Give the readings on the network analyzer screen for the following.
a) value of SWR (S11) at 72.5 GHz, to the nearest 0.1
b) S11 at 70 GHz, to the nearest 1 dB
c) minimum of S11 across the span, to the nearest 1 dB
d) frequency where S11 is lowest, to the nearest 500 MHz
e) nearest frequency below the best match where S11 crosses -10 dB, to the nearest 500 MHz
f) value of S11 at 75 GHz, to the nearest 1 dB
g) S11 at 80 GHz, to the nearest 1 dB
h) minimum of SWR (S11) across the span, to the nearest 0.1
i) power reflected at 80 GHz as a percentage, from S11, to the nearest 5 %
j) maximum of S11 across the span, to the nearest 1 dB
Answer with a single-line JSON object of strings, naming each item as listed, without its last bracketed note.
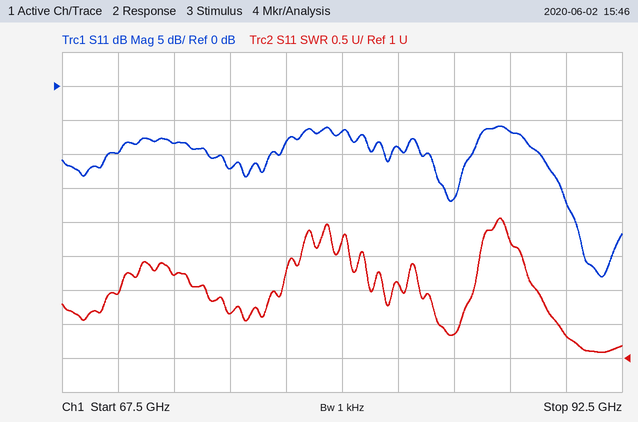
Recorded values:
{"value of SWR (S11) at 72.5 GHz, to the nearest 0.1": "2.2", "S11 at 70 GHz, to the nearest 1 dB": "-10 dB", "minimum of S11 across the span, to the nearest 1 dB": "-28 dB", "frequency where S11 is lowest, to the nearest 500 MHz": "91.5 GHz", "nearest frequency below the best match where S11 crosses -10 dB, to the nearest 500 MHz": "89.0 GHz", "value of S11 at 75 GHz, to the nearest 1 dB": "-12 dB", "S11 at 80 GHz, to the nearest 1 dB": "-7 dB", "minimum of SWR (S11) across the span, to the nearest 0.1": "1.1", "power reflected at 80 GHz as a percentage, from S11, to the nearest 5 %": "20 %", "maximum of S11 across the span, to the nearest 1 dB": "-6 dB"}
